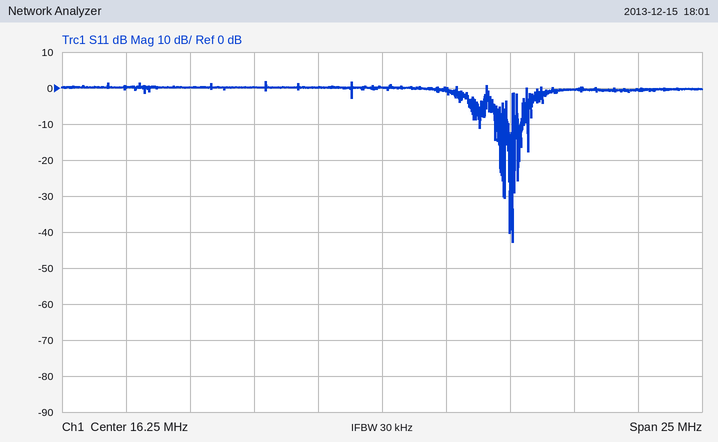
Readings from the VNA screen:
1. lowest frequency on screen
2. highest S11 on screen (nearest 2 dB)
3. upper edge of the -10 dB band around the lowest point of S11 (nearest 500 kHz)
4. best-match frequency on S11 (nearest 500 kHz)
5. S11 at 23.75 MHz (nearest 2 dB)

3.75 MHz
2 dB
21.5 MHz
21.5 MHz
0 dB
